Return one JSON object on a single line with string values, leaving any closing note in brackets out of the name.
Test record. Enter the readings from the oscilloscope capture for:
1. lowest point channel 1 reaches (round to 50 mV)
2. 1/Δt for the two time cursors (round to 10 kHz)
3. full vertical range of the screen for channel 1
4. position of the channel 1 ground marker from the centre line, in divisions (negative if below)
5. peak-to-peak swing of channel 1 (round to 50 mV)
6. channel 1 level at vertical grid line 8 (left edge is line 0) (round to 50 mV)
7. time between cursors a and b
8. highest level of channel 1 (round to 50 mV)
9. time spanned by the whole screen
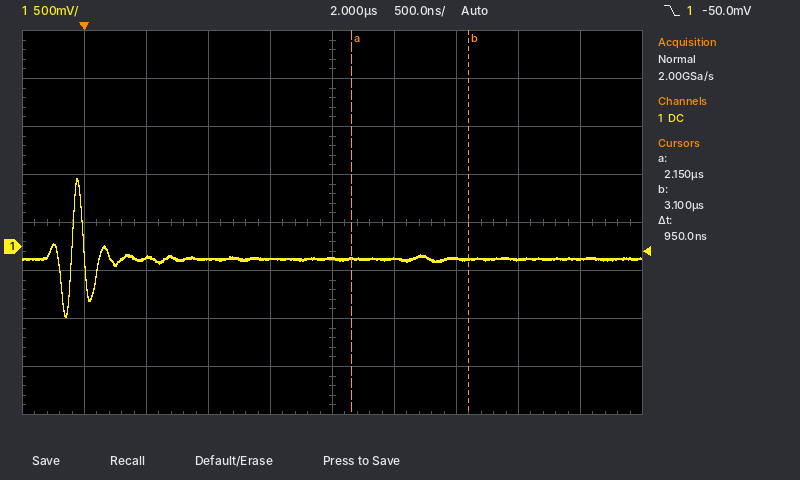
{"lowest point channel 1 reaches": "-750 mV", "1/Δt for the two time cursors": "1.05 MHz", "full vertical range of the screen for channel 1": "4 V", "position of the channel 1 ground marker from the centre line, in divisions": "-0.5 div", "peak-to-peak swing of channel 1": "1.45 V", "channel 1 level at vertical grid line 8 (left edge is line 0)": "-150 mV", "time between cursors a and b": "950 ns", "highest level of channel 1": "700 mV", "time spanned by the whole screen": "5 µs"}
